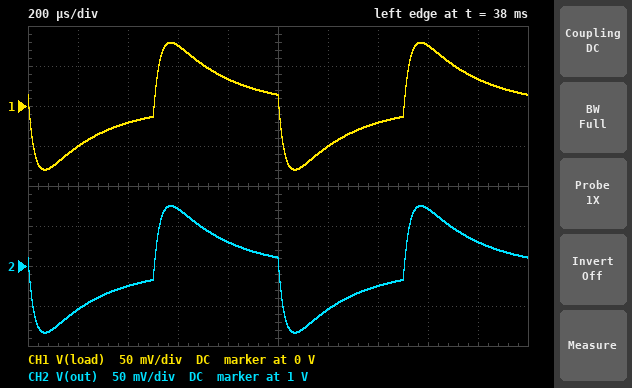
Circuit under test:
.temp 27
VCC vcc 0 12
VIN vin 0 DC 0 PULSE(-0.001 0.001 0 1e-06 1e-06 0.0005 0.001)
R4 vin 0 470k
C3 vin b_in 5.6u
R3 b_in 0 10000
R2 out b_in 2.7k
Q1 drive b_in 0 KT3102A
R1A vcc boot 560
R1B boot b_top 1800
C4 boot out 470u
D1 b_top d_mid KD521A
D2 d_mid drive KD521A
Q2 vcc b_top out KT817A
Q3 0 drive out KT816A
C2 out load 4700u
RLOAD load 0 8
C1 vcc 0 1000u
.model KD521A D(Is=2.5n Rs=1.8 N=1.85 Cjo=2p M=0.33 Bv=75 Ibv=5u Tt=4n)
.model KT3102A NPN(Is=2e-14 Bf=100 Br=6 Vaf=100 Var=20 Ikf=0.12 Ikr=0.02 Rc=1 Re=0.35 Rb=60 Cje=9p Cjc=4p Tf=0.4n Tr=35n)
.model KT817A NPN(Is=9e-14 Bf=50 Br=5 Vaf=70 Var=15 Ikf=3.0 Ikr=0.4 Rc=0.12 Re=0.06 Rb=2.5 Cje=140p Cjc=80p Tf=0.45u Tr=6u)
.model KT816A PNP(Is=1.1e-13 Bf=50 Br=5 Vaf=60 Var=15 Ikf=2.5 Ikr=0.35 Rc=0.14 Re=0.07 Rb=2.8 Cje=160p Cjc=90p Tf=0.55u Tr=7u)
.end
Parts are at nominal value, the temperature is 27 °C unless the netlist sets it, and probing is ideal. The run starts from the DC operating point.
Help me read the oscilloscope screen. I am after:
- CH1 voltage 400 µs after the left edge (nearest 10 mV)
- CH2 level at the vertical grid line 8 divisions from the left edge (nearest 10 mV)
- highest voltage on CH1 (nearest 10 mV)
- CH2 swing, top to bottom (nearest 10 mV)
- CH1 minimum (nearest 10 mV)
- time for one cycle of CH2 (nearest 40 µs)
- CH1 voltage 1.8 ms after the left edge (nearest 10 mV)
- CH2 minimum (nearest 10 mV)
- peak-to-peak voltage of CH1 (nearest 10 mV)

-20 mV
1.07 V
80 mV
160 mV
-80 mV
1.00 ms
30 mV
920 mV
160 mV
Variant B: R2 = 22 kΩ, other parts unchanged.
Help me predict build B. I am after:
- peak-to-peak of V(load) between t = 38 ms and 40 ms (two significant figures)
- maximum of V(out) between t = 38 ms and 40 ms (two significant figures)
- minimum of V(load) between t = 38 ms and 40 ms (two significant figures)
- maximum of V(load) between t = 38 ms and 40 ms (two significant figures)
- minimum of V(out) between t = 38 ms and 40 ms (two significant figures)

100 mV
3.0 V
-49 mV
51 mV
2.9 V
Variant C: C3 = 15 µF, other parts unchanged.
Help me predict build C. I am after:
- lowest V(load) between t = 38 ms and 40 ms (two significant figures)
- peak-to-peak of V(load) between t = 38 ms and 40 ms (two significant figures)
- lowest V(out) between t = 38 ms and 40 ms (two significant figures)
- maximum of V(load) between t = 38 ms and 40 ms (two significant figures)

-65 mV
130 mV
930 mV
66 mV
